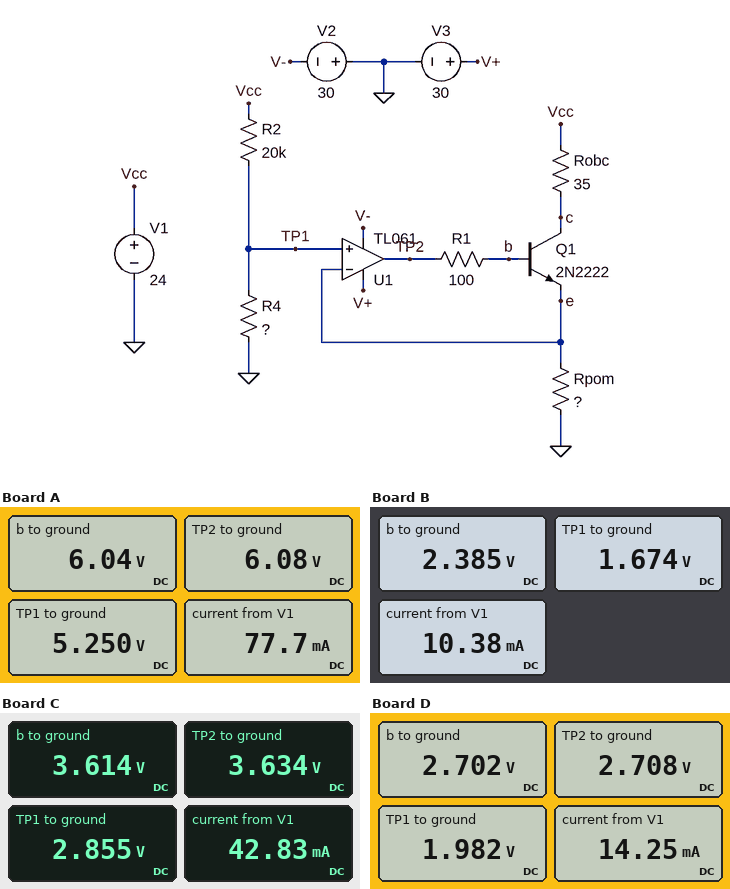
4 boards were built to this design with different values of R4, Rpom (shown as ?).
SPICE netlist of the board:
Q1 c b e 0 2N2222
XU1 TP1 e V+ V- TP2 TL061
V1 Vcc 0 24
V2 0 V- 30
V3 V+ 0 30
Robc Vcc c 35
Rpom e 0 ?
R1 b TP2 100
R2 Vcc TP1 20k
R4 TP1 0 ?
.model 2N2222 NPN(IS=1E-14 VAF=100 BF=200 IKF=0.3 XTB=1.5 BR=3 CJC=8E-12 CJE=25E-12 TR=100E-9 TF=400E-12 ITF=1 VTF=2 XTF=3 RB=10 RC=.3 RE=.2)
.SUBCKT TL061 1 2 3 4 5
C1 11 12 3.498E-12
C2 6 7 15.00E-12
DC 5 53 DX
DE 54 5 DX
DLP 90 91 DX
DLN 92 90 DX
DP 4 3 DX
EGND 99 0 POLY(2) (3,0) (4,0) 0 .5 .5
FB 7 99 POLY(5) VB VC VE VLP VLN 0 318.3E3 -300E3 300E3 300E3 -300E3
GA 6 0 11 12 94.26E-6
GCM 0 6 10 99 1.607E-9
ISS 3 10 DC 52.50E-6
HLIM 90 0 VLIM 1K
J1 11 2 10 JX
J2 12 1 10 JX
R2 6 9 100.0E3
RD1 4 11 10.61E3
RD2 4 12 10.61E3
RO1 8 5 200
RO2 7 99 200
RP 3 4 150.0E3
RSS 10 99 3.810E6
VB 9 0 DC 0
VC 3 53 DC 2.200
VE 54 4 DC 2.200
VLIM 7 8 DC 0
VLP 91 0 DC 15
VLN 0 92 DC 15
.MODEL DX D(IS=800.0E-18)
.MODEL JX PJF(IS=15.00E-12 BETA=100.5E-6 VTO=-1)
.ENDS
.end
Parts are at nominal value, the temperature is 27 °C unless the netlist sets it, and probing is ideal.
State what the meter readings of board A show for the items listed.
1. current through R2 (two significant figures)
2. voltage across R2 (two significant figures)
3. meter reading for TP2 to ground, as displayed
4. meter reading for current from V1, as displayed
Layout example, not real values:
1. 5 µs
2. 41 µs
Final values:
1. 940 µA
2. 19 V
3. 6.08 V
4. 77.7 mA
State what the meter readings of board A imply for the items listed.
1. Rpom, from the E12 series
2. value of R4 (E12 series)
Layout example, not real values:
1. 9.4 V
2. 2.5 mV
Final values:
1. 68 Ω
2. 5.6 kΩ
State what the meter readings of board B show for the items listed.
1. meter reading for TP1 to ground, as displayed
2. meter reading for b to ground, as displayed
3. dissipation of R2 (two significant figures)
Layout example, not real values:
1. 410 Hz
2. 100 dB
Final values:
1. 1.674 V
2. 2.385 V
3. 25 mW
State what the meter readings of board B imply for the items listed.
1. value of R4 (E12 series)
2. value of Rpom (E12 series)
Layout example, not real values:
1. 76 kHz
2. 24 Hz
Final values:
1. 1.5 kΩ
2. 180 Ω
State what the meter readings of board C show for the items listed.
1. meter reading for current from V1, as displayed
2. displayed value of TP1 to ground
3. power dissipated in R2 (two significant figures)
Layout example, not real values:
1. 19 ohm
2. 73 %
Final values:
1. 42.83 mA
2. 2.855 V
3. 22 mW
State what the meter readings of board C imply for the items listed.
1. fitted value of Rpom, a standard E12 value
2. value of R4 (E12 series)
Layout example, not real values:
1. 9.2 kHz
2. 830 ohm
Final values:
1. 68 Ω
2. 2.7 kΩ
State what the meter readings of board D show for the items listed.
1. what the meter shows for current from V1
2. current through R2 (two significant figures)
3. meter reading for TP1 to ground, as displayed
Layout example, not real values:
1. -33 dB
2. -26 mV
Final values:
1. 14.25 mA
2. 1.1 mA
3. 1.982 V
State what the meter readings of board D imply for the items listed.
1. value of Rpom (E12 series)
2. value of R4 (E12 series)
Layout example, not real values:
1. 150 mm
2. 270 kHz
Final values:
1. 150 Ω
2. 1.8 kΩ
